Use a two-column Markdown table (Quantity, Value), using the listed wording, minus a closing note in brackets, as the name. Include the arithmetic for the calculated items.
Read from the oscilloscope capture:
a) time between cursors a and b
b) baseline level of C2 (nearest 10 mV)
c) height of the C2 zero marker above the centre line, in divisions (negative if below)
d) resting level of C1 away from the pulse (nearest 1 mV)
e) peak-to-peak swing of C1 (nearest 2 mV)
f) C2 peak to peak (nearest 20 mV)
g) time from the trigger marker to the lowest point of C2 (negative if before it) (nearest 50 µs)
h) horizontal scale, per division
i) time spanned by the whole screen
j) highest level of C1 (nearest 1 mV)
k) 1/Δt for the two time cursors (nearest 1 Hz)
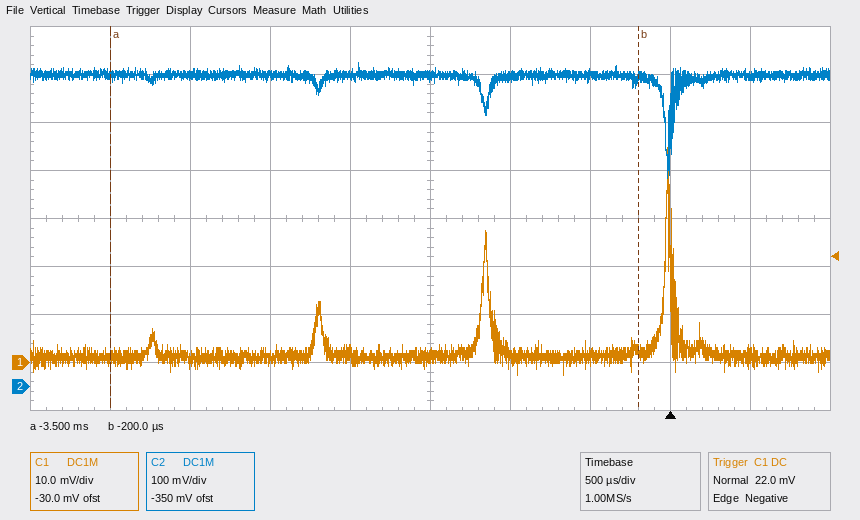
| Quantity | Value |
|---|---|
| time between cursors a and b | -200 µs − (-3.5 ms) = 3.30 ms |
| baseline level of C2 | 650 mV |
| height of the C2 zero marker above the centre line, in divisions | -3.5 div |
| resting level of C1 away from the pulse | 1 mV |
| peak-to-peak swing of C1 | 48 mV |
| C2 peak to peak | 240 mV |
| time from the trigger marker to the lowest point of C2 (negative if before it) | 0 µs |
| horizontal scale, per division | 500 µs |
| time spanned by the whole screen | 5 ms |
| highest level of C1 | 45 mV |
| 1/Δt for the two time cursors | 1 / 3.30 ms ≈ 303 Hz |
